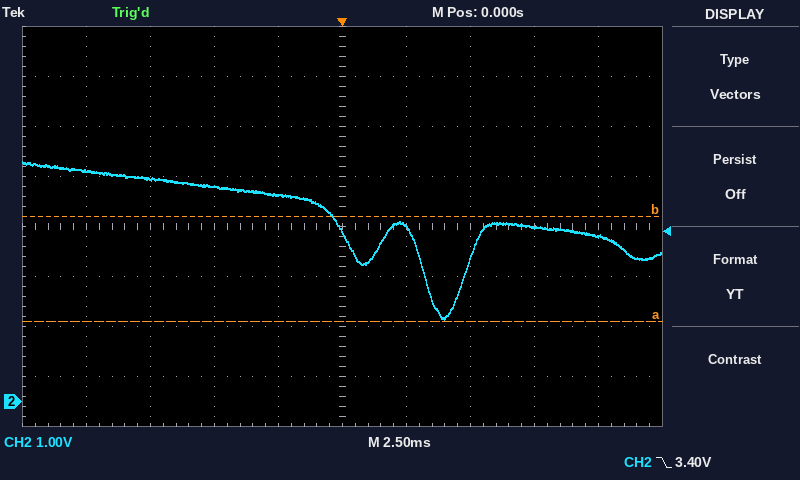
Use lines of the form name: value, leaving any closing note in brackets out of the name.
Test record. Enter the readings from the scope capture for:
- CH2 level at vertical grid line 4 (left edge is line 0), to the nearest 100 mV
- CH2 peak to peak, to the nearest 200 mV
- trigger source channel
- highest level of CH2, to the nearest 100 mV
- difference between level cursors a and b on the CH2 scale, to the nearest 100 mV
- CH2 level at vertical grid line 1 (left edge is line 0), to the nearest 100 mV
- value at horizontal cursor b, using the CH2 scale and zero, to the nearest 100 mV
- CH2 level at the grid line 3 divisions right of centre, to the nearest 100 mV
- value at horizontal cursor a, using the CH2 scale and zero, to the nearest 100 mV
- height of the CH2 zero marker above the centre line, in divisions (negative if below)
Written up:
CH2 level at vertical grid line 4 (left edge is line 0), to the nearest 100 mV: 4.1 V
CH2 peak to peak, to the nearest 200 mV: 3.2 V
trigger source channel: CH2
highest level of CH2, to the nearest 100 mV: 4.8 V
difference between level cursors a and b on the CH2 scale, to the nearest 100 mV: 2.1 V
CH2 level at vertical grid line 1 (left edge is line 0), to the nearest 100 mV: 4.6 V
value at horizontal cursor b, using the CH2 scale and zero, to the nearest 100 mV: 3.7 V
CH2 level at the grid line 3 divisions right of centre, to the nearest 100 mV: 3.5 V
value at horizontal cursor a, using the CH2 scale and zero, to the nearest 100 mV: 1.6 V
height of the CH2 zero marker above the centre line, in divisions: -3.5 div
